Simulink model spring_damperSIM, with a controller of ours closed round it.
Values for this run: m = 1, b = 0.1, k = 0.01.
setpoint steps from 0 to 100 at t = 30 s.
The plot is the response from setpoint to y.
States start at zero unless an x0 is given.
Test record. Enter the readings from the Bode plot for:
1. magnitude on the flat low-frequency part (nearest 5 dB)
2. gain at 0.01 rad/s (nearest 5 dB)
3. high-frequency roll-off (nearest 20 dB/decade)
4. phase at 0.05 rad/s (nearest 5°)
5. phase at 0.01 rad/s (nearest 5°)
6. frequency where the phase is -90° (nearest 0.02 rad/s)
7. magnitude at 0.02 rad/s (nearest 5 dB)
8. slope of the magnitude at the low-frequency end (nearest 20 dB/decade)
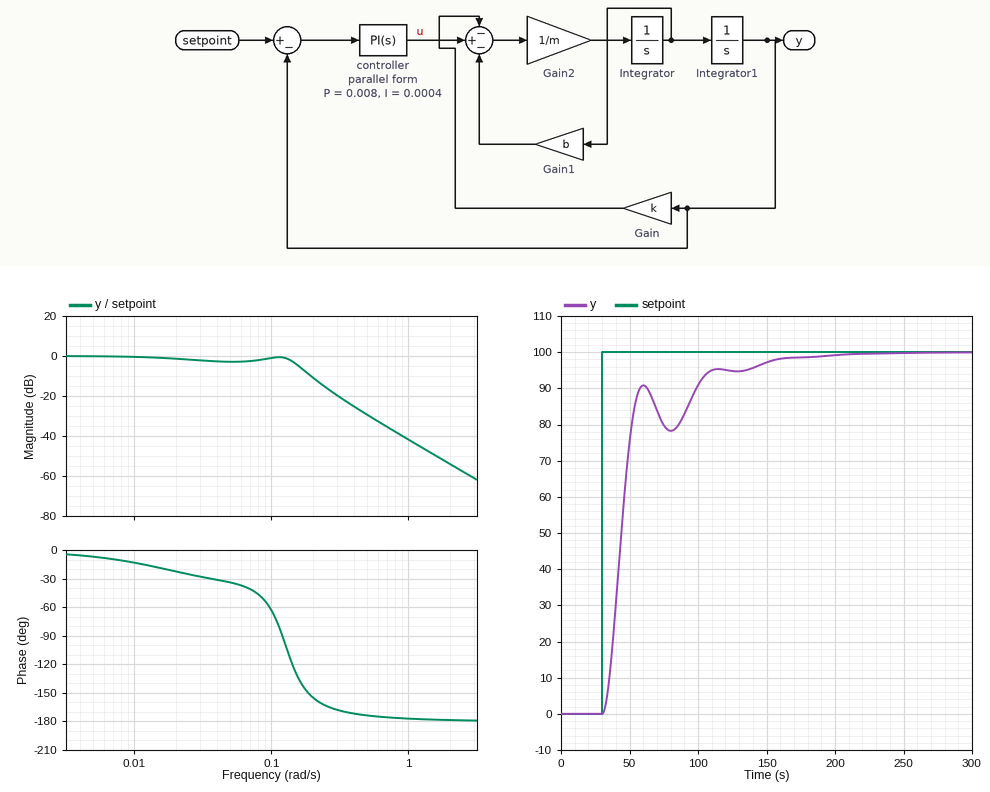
0 dB
0 dB
-40 dB/decade
-35°
-15°
0.12 rad/s
0 dB
0 dB/decade
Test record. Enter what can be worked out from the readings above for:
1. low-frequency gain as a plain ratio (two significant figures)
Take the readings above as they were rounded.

1.0
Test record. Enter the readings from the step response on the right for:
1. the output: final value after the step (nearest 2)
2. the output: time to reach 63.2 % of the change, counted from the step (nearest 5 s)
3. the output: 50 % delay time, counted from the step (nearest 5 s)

100
15 s
15 s
